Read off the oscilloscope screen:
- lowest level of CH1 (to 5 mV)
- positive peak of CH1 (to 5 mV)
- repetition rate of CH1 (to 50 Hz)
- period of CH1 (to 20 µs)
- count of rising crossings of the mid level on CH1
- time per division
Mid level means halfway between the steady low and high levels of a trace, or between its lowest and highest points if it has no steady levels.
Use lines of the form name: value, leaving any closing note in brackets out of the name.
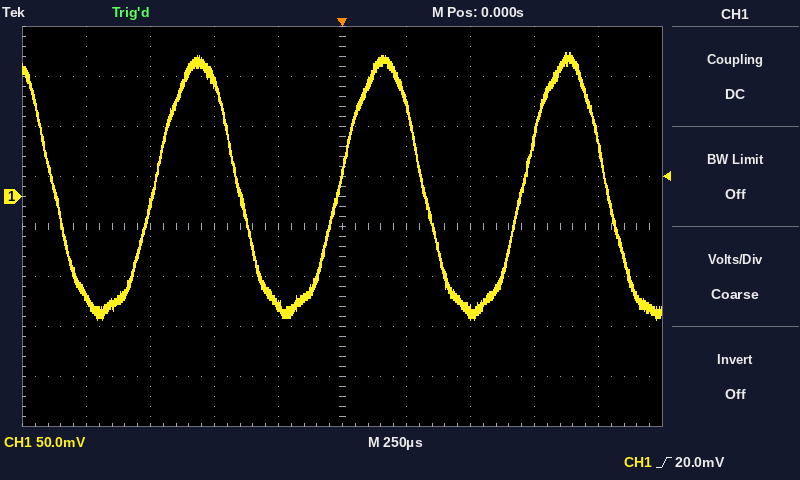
lowest level of CH1: -125 mV
positive peak of CH1: 145 mV
repetition rate of CH1: 1.40 kHz
period of CH1: 720 µs
count of rising crossings of the mid level on CH1: 3
time per division: 250 µs
